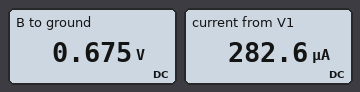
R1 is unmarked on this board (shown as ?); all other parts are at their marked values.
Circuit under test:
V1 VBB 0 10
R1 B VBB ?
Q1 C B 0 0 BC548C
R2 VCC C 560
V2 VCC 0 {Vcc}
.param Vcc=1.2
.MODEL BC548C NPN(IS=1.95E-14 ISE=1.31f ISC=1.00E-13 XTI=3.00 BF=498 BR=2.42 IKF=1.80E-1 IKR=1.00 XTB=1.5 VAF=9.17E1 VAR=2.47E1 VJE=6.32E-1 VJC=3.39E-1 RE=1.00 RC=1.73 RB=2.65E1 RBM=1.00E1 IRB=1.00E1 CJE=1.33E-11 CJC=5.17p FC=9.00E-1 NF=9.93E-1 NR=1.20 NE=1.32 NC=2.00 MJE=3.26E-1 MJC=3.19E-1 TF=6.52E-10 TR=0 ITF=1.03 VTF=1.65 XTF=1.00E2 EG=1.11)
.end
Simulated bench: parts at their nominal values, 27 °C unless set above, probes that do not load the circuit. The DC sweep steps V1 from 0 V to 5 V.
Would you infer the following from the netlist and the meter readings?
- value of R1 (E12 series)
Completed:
33 kΩ
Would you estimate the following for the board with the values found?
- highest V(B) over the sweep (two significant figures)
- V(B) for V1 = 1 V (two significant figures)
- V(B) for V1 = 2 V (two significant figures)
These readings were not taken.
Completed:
670 mV
660 mV
660 mV
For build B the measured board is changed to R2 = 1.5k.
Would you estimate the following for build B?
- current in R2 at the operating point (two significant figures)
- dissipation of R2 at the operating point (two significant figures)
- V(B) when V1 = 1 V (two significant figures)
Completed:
870 µA
1.1 mW
630 mV
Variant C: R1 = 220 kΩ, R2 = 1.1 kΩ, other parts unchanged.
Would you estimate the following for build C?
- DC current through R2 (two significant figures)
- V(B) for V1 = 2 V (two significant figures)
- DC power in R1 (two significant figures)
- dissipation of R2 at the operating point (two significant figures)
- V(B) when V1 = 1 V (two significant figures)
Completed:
1.1 mA
640 mV
400 µW
1.4 mW
630 mV
